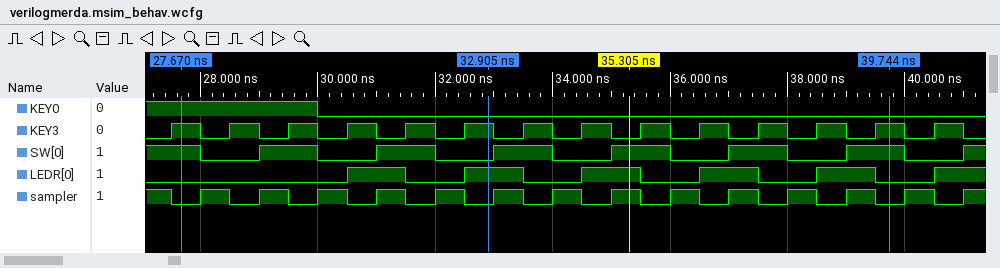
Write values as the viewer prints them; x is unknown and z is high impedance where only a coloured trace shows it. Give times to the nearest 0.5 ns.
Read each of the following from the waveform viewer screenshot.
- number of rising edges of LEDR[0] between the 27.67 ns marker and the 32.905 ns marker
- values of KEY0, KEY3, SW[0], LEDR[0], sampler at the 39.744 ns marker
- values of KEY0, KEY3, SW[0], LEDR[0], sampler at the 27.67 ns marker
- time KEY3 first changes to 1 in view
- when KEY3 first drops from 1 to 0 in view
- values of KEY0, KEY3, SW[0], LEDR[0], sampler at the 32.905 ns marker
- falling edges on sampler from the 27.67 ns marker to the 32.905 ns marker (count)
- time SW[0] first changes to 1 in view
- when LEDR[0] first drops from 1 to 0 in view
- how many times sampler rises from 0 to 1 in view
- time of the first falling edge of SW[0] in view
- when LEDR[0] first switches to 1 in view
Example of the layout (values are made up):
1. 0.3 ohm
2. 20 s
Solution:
1. 2
2. KEY0=0, KEY3=1, SW[0]=1, LEDR[0]=0, sampler=0
3. KEY0=1, KEY3=1, SW[0]=1, LEDR[0]=0, sampler=0
4. 27.5 ns
5. 28 ns
6. KEY0=0, KEY3=1, SW[0]=0, LEDR[0]=1, sampler=0
7. 5
8. 29 ns
9. 31.5 ns
10. 14
11. 28 ns
12. 30.5 ns
